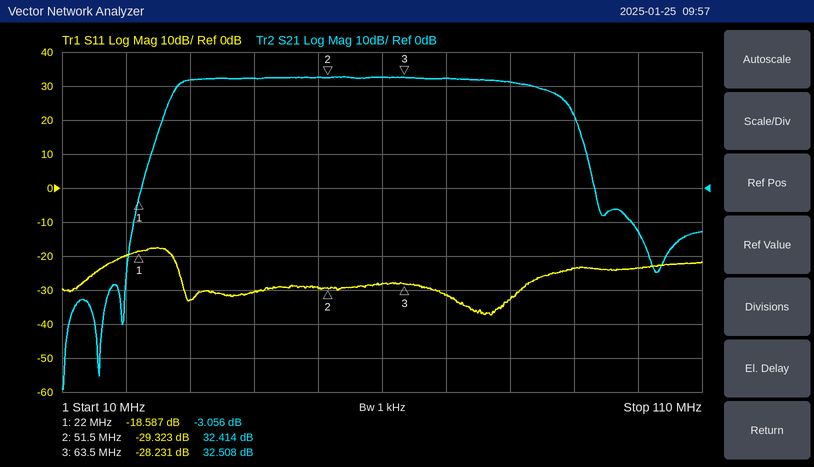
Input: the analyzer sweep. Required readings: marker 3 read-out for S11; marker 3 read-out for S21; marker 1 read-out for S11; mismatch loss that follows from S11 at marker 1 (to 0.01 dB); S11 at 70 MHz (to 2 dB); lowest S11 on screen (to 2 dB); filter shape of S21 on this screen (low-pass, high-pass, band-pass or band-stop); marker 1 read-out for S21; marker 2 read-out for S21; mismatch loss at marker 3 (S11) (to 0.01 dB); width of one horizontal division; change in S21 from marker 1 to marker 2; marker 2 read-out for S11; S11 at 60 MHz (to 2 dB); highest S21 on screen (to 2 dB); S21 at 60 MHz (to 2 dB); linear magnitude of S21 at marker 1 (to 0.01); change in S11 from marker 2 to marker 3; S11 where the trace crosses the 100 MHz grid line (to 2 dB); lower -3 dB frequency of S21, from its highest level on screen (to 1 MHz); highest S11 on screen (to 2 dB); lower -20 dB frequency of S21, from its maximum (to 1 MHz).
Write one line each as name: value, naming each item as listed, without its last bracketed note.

marker 3 read-out for S11: -28.231 dB
marker 3 read-out for S21: 32.508 dB
marker 1 read-out for S11: -18.587 dB
mismatch loss that follows from S11 at marker 1: 0.06 dB
S11 at 70 MHz: -32 dB
lowest S11 on screen: -38 dB
filter shape of S21 on this screen: band-pass
marker 1 read-out for S21: -3.056 dB
marker 2 read-out for S21: 32.414 dB
mismatch loss at marker 3 (S11): 0.01 dB
width of one horizontal division: 10 MHz
change in S21 from marker 1 to marker 2: 35.470 dB
marker 2 read-out for S11: -29.323 dB
S11 at 60 MHz: -28 dB
highest S21 on screen: 32 dB
S21 at 60 MHz: 32 dB
linear magnitude of S21 at marker 1: 0.70
change in S11 from marker 2 to marker 3: 1.092 dB
S11 where the trace crosses the 100 MHz grid line: -24 dB
lower -3 dB frequency of S21, from its highest level on screen: 28 MHz
highest S11 on screen: -18 dB
lower -20 dB frequency of S21, from its maximum: 24 MHz
